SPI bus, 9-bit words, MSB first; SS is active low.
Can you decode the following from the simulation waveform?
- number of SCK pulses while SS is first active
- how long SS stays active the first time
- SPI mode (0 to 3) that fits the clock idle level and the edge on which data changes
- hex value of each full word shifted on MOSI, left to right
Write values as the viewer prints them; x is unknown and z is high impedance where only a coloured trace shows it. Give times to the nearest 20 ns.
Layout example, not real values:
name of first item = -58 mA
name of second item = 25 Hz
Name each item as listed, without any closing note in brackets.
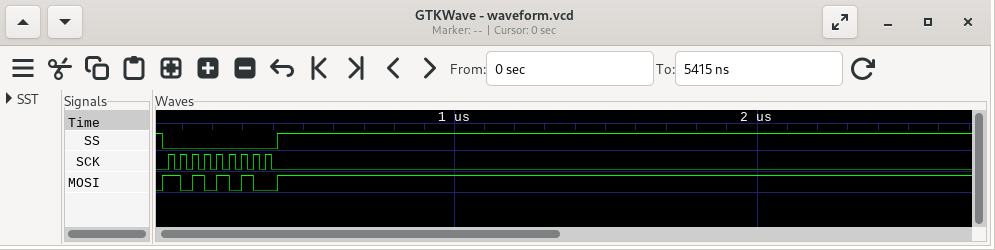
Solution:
number of SCK pulses while SS is first active = 9
how long SS stays active the first time = 380 ns
SPI mode (0 to 3) that fits the clock idle level and the edge on which data changes = 1
hex value of each full word shifted on MOSI, left to right = 154
